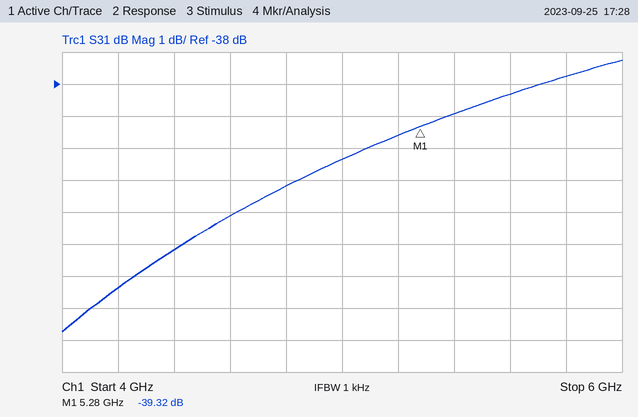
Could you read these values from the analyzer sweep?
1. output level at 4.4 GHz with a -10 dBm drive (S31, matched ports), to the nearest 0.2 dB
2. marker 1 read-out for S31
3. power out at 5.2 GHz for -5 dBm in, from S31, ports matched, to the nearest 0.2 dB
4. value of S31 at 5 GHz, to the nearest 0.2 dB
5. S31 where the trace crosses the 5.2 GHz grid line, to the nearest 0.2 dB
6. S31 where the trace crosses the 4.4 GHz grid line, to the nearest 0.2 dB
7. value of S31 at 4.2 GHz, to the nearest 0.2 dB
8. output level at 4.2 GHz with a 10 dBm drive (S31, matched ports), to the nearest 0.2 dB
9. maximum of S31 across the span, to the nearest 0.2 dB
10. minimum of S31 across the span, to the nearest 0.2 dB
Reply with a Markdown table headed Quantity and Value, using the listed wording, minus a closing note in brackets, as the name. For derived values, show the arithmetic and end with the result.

| Quantity | Value |
|---|---|
| output level at 4.4 GHz with a -10 dBm drive (S31, matched ports), to the nearest 0.2 dB | -10 dBm + (-43.2 dB) = -53.2 dBm |
| marker 1 read-out for S31 | -39.32 dB |
| power out at 5.2 GHz for -5 dBm in, from S31, ports matched, to the nearest 0.2 dB | -5 dBm + (-39.6 dB) = -44.6 dBm |
| value of S31 at 5 GHz, to the nearest 0.2 dB | -40.4 dB |
| S31 where the trace crosses the 5.2 GHz grid line, to the nearest 0.2 dB | -39.6 dB |
| S31 where the trace crosses the 4.4 GHz grid line, to the nearest 0.2 dB | -43.2 dB |
| value of S31 at 4.2 GHz, to the nearest 0.2 dB | -44.4 dB |
| output level at 4.2 GHz with a 10 dBm drive (S31, matched ports), to the nearest 0.2 dB | 10 dBm + (-44.4 dB) = -34.4 dBm |
| maximum of S31 across the span, to the nearest 0.2 dB | -37.2 dB |
| minimum of S31 across the span, to the nearest 0.2 dB | -45.8 dB |
